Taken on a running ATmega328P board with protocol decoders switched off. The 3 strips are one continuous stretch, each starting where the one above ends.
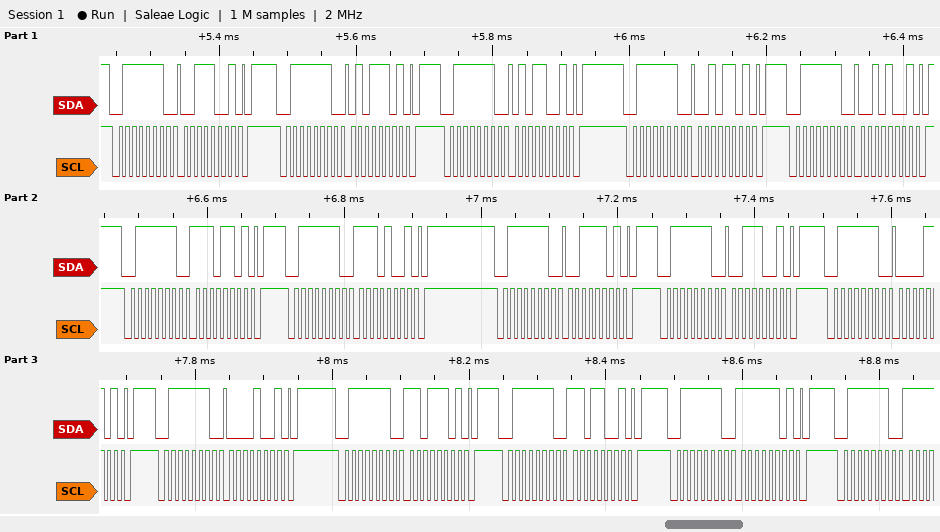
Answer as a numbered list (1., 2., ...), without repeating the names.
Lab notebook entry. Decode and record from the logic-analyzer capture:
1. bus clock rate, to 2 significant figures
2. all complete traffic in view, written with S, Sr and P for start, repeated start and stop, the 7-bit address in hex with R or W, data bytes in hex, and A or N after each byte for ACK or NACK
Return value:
1. 100 kHz
2. S 3FW A 39 A P S 3FW A 5D A P S 3FW A 59 A P S 3FW A 2D A P S 3FW A 29 A P S 3FW A ED A P S 3FW A E9 A P S 3FW A 3D A P S 3FW A 39 A P S 3FW A 0D A P S 3FW A 09 A P S 3FW A DD A P S 3FW A D9 A P S 3FW A FD A P S 3FW A
